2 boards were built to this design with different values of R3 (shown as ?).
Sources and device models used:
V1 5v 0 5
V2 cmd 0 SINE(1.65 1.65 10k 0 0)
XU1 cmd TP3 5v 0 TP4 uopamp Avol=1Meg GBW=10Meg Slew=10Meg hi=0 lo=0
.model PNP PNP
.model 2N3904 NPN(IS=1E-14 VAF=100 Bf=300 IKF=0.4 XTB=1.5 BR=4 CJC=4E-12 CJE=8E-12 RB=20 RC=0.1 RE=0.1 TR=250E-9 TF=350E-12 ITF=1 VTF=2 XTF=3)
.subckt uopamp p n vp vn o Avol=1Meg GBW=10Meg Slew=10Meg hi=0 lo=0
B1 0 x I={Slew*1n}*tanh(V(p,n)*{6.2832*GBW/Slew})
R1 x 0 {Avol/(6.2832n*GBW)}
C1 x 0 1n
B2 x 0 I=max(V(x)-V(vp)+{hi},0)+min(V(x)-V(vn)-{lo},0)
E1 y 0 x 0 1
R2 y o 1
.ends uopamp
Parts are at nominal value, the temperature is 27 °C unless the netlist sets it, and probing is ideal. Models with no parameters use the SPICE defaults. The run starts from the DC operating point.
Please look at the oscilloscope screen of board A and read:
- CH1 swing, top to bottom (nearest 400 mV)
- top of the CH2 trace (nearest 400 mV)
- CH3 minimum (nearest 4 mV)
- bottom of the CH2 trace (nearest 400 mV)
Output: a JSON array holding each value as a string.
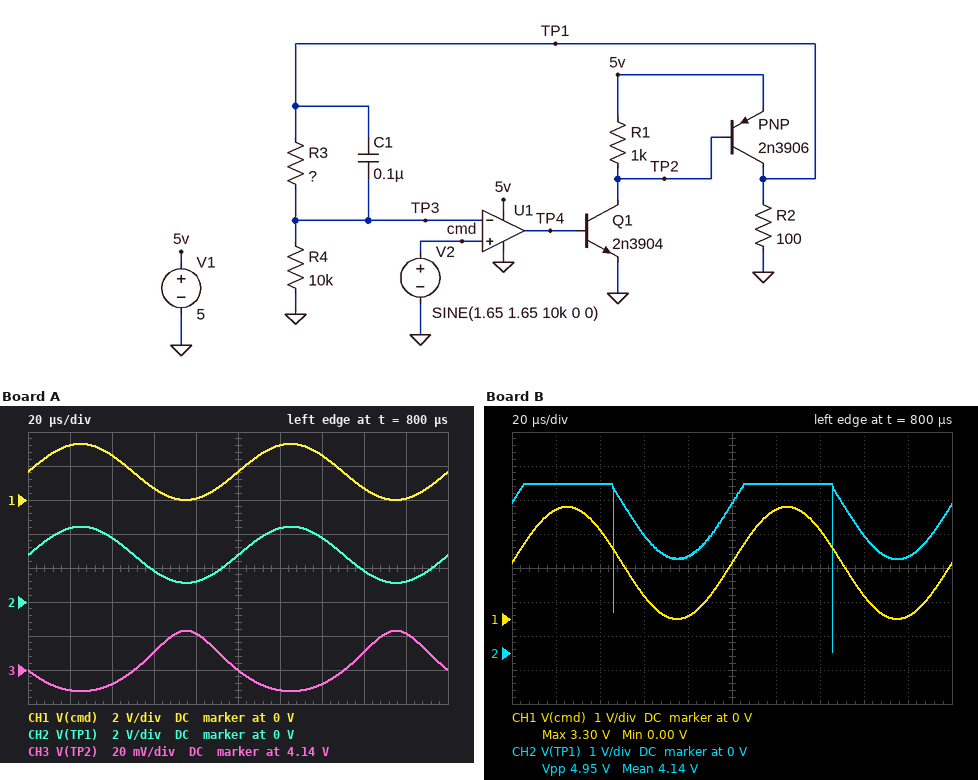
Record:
["3.2 V", "4.4 V", "4.128 V", "1.2 V"]
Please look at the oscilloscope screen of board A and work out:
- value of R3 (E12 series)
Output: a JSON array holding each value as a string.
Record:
["6.8 kΩ"]
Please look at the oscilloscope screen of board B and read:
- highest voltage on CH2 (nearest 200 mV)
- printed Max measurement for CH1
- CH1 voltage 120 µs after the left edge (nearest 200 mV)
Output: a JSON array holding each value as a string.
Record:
["5.0 V", "3.30 V", "3.2 V"]
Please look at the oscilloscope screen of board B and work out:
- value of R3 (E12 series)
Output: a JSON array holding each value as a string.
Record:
["18 kΩ"]
